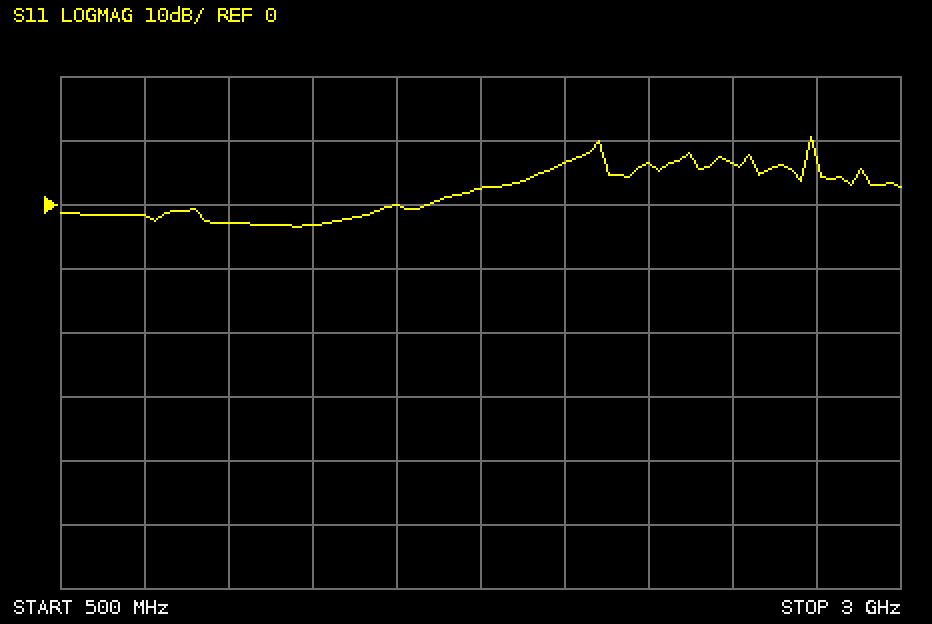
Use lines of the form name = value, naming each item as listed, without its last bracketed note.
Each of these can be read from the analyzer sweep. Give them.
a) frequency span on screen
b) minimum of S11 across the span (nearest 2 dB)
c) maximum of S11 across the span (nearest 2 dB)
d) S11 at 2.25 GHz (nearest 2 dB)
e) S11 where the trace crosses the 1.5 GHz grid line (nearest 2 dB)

frequency span on screen = 2.5 GHz
minimum of S11 across the span = -4 dB
maximum of S11 across the span = 10 dB
S11 at 2.25 GHz = 6 dB
S11 where the trace crosses the 1.5 GHz grid line = 0 dB
